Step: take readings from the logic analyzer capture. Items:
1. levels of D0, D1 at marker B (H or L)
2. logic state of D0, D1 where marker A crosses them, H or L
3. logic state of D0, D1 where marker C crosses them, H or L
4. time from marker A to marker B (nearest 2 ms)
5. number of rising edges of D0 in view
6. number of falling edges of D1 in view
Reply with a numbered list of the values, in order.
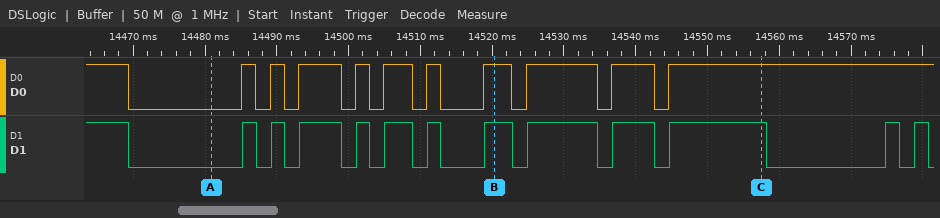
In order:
1. D0=H, D1=H
2. D0=L, D1=L
3. D0=H, D1=H
4. 40 ms
5. 10
6. 13
